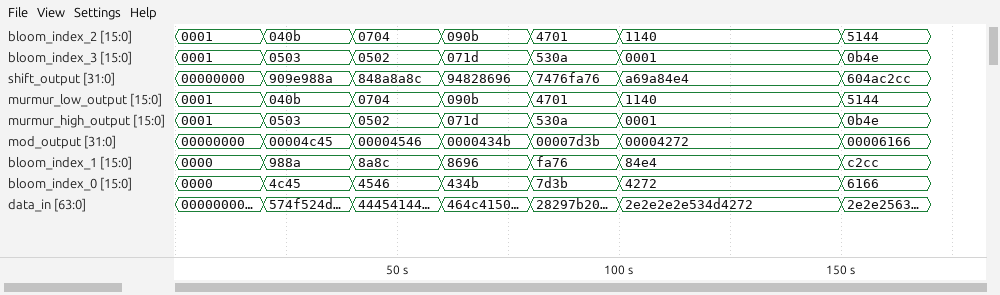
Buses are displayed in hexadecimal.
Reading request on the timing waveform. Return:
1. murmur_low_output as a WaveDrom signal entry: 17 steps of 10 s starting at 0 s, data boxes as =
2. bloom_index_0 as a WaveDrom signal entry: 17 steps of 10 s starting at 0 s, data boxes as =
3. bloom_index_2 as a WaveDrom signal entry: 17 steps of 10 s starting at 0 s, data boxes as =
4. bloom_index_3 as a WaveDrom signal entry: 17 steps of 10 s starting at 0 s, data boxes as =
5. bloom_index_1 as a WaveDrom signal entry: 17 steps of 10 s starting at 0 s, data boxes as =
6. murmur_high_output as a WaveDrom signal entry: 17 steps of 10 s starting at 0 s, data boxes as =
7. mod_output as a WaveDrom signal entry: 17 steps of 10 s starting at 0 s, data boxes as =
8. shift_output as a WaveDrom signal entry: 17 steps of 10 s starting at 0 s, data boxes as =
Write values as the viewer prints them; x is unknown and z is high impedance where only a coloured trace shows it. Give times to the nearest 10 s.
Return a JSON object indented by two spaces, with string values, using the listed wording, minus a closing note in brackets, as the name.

{
  "murmur_low_output as a WaveDrom signal entry: 17 steps of 10 s starting at 0 s, data boxes as =": "{name: 'murmur_low_output', wave: '=.=.=.=.=.=....=.', data: '0001 040b 0704 090b 4701 1140 5144'}",
  "bloom_index_0 as a WaveDrom signal entry: 17 steps of 10 s starting at 0 s, data boxes as =": "{name: 'bloom_index_0', wave: '=.=.=.=.=.=....=.', data: '0000 4c45 4546 434b 7d3b 4272 6166'}",
  "bloom_index_2 as a WaveDrom signal entry: 17 steps of 10 s starting at 0 s, data boxes as =": "{name: 'bloom_index_2', wave: '=.=.=.=.=.=....=.', data: '0001 040b 0704 090b 4701 1140 5144'}",
  "bloom_index_3 as a WaveDrom signal entry: 17 steps of 10 s starting at 0 s, data boxes as =": "{name: 'bloom_index_3', wave: '=.=.=.=.=.=....=.', data: '0001 0503 0502 071d 530a 0001 0b4e'}",
  "bloom_index_1 as a WaveDrom signal entry: 17 steps of 10 s starting at 0 s, data boxes as =": "{name: 'bloom_index_1', wave: '=.=.=.=.=.=....=.', data: '0000 988a 8a8c 8696 fa76 84e4 c2cc'}",
  "murmur_high_output as a WaveDrom signal entry: 17 steps of 10 s starting at 0 s, data boxes as =": "{name: 'murmur_high_output', wave: '=.=.=.=.=.=....=.', data: '0001 0503 0502 071d 530a 0001 0b4e'}",
  "mod_output as a WaveDrom signal entry: 17 steps of 10 s starting at 0 s, data boxes as =": "{name: 'mod_output', wave: '=.=.=.=.=.=....=.', data: '00000000 00004c45 00004546 0000434b 00007d3b 00004272 00006166'}",
  "shift_output as a WaveDrom signal entry: 17 steps of 10 s starting at 0 s, data boxes as =": "{name: 'shift_output', wave: '=.=.=.=.=.=....=.', data: '00000000 909e988a 848a8a8c 94828696 7476fa76 a69a84e4 604ac2cc'}"
}
